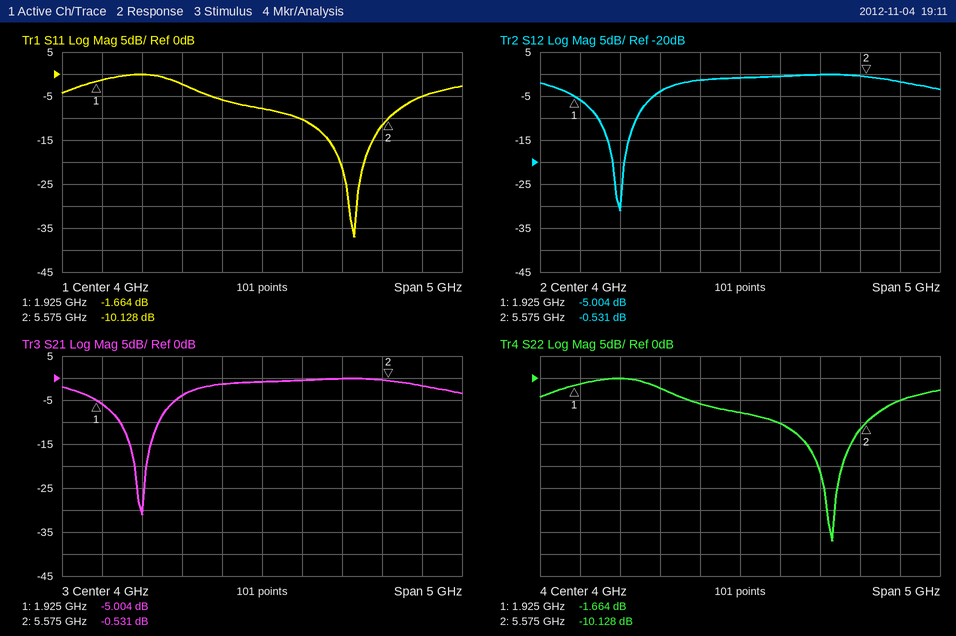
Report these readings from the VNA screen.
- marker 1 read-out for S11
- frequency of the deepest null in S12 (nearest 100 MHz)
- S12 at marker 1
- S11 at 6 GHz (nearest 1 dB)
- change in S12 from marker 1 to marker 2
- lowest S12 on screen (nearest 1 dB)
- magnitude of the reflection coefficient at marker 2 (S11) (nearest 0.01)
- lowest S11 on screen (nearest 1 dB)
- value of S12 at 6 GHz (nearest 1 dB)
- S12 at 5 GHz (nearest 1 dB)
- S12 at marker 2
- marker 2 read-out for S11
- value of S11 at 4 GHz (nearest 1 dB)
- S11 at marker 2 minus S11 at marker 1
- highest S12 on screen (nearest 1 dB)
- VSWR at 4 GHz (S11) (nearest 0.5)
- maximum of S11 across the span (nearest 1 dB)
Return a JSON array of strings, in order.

["-1.664 dB", "2.5 GHz", "-5.004 dB", "-5 dB", "4.473 dB", "-31 dB", "0.31", "-37 dB", "-2 dB", "0 dB", "-0.531 dB", "-10.128 dB", "-8 dB", "-8.464 dB", "0 dB", "2.5", "0 dB"]
